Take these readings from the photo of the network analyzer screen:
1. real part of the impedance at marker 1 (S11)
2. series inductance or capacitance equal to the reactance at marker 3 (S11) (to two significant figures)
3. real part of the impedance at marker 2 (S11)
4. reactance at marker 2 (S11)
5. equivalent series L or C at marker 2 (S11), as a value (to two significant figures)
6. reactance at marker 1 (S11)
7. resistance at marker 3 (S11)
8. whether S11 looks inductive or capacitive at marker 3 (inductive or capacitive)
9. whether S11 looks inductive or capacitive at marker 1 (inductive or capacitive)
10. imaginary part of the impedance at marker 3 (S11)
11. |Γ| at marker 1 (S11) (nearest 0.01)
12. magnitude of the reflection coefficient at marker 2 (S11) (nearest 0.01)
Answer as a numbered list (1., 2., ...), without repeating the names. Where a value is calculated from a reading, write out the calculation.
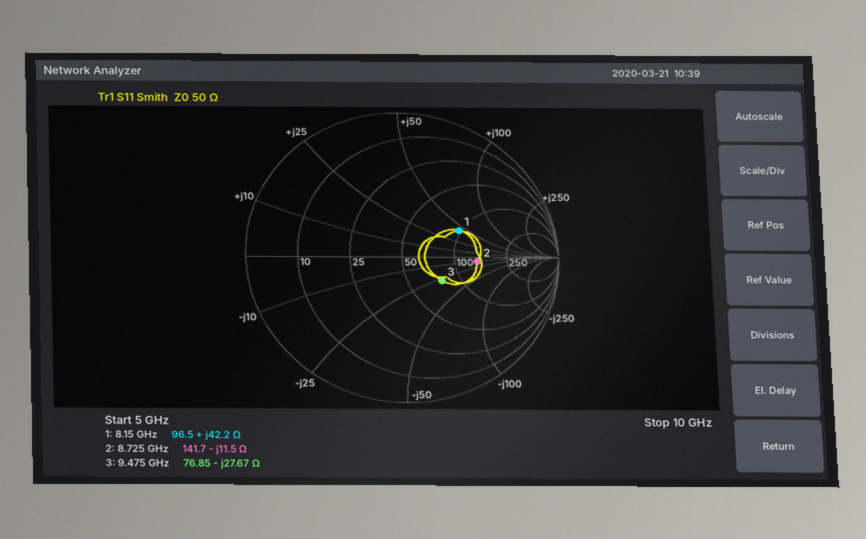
1. 96.5 Ω
2. C = 1/(2π × 9.475 GHz × 27.67 Ω) ≈ 607 fF, so 610 fF to two significant figures
3. 141.7 Ω
4. -11.5 Ω
5. C = 1/(2π × 8.725 GHz × 11.5 Ω) ≈ 1.6 pF
6. +42.2 Ω
7. 76.85 Ω
8. capacitive
9. inductive
10. -27.67 Ω
11. 0.41
12. 0.48
